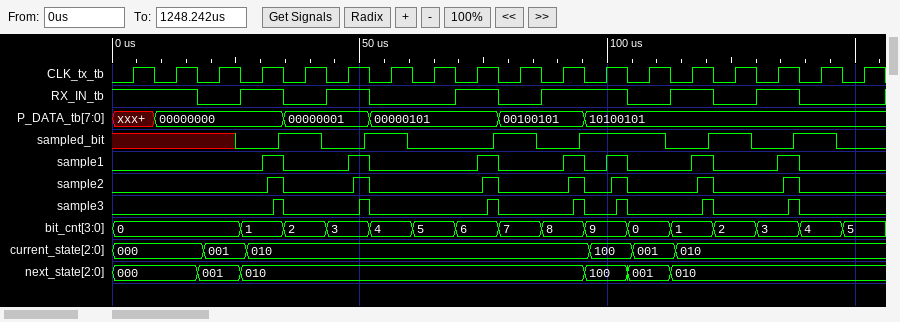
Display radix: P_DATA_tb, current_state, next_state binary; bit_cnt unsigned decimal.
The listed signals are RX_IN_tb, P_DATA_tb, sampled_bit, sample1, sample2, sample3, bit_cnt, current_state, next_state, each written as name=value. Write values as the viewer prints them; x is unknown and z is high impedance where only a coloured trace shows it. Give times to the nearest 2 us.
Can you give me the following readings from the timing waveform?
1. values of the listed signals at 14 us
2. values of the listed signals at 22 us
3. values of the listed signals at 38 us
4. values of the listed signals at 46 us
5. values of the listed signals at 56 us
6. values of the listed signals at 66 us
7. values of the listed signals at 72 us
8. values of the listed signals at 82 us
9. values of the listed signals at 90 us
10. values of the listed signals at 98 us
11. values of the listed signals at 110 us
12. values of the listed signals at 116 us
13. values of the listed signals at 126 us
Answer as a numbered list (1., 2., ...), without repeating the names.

1. RX_IN_tb=1, P_DATA_tb=00000000, sampled_bit=x, sample1=0, sample2=0, sample3=0, bit_cnt=0, current_state=000, next_state=000
2. RX_IN_tb=0, P_DATA_tb=00000000, sampled_bit=x, sample1=0, sample2=0, sample3=0, bit_cnt=0, current_state=001, next_state=001
3. RX_IN_tb=0, P_DATA_tb=00000001, sampled_bit=1, sample1=0, sample2=0, sample3=0, bit_cnt=2, current_state=010, next_state=010
4. RX_IN_tb=1, P_DATA_tb=00000001, sampled_bit=0, sample1=0, sample2=0, sample3=0, bit_cnt=3, current_state=010, next_state=010
5. RX_IN_tb=0, P_DATA_tb=00000101, sampled_bit=1, sample1=0, sample2=0, sample3=0, bit_cnt=4, current_state=010, next_state=010
6. RX_IN_tb=0, P_DATA_tb=00000101, sampled_bit=0, sample1=0, sample2=0, sample3=0, bit_cnt=5, current_state=010, next_state=010
7. RX_IN_tb=1, P_DATA_tb=00000101, sampled_bit=0, sample1=0, sample2=0, sample3=0, bit_cnt=6, current_state=010, next_state=010
8. RX_IN_tb=0, P_DATA_tb=00100101, sampled_bit=1, sample1=0, sample2=0, sample3=0, bit_cnt=7, current_state=010, next_state=010
9. RX_IN_tb=1, P_DATA_tb=00100101, sampled_bit=0, sample1=0, sample2=0, sample3=0, bit_cnt=8, current_state=010, next_state=010
10. RX_IN_tb=1, P_DATA_tb=10100101, sampled_bit=1, sample1=0, sample2=0, sample3=0, bit_cnt=9, current_state=100, next_state=100
11. RX_IN_tb=0, P_DATA_tb=10100101, sampled_bit=1, sample1=0, sample2=0, sample3=0, bit_cnt=0, current_state=001, next_state=001
12. RX_IN_tb=1, P_DATA_tb=10100101, sampled_bit=0, sample1=0, sample2=0, sample3=0, bit_cnt=1, current_state=010, next_state=010
13. RX_IN_tb=0, P_DATA_tb=10100101, sampled_bit=1, sample1=0, sample2=0, sample3=0, bit_cnt=2, current_state=010, next_state=010
